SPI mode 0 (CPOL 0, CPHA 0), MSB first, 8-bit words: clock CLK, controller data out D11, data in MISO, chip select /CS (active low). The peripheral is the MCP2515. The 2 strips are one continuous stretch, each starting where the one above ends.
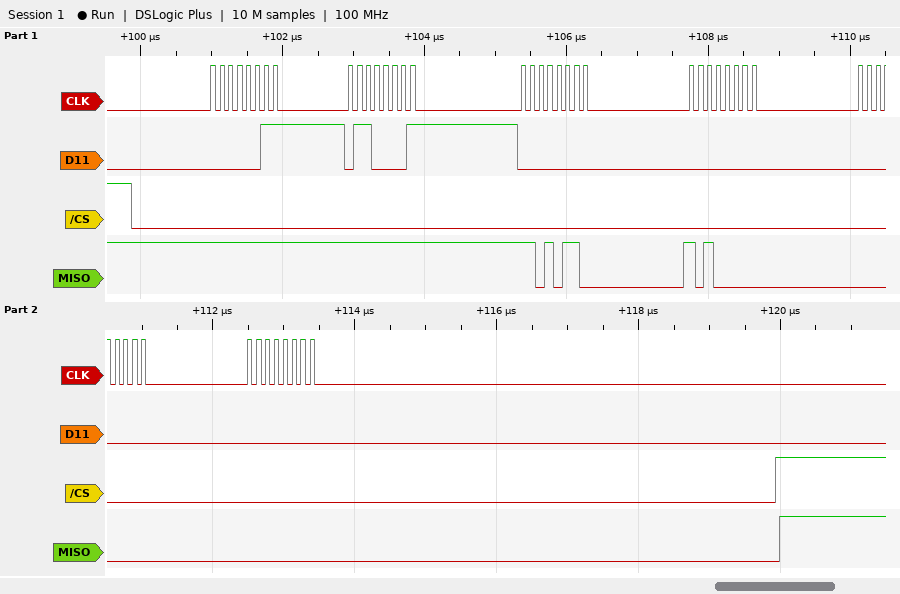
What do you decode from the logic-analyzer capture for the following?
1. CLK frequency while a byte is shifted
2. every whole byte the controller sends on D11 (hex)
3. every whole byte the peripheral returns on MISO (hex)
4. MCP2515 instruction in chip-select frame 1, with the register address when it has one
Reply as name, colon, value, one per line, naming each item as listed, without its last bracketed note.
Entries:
CLK frequency while a byte is shifted: 8 MHz
every whole byte the controller sends on D11: 03 61 00 00 00 00
every whole byte the peripheral returns on MISO: FF FF D6 A0 00 00
MCP2515 instruction in chip-select frame 1, with the register address when it has one: READ 0x61
